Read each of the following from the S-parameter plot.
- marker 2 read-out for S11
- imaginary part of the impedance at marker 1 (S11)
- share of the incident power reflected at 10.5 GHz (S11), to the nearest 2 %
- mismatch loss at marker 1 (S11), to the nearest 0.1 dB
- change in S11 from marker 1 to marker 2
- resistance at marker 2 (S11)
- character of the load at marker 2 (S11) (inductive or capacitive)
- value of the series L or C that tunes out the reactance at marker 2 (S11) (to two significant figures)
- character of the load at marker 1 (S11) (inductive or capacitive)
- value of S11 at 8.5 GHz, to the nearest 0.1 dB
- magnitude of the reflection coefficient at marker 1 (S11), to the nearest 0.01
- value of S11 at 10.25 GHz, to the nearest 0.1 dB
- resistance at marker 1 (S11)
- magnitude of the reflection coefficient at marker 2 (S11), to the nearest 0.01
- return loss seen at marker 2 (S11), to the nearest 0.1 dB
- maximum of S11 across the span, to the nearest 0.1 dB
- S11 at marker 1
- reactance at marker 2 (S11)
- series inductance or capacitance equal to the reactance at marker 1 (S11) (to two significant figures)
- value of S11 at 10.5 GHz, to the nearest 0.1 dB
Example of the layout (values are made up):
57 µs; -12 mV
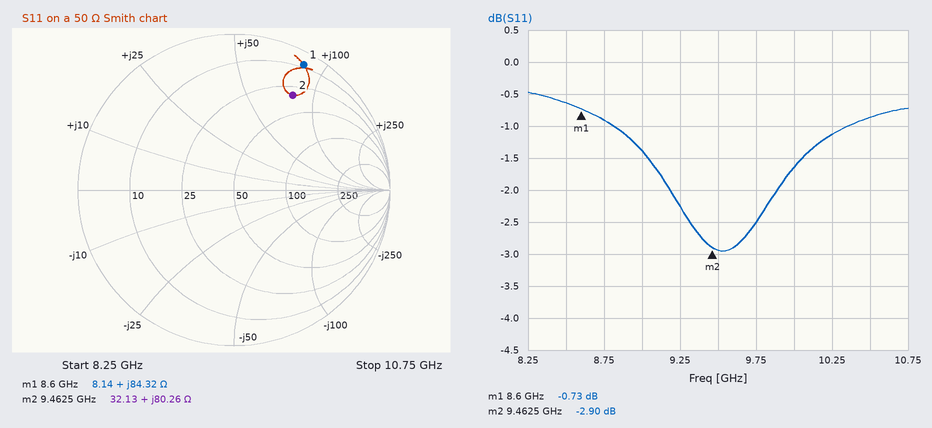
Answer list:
-2.90 dB; +84.32 Ω; 82 %; 8.1 dB; -2.17 dB; 32.13 Ω; inductive; 210 fF; inductive; -0.6 dB; 0.92; -1.1 dB; 8.14 Ω; 0.72; 2.9 dB; -0.5 dB; -0.73 dB; +80.26 Ω; 1.6 nH; -0.9 dB
